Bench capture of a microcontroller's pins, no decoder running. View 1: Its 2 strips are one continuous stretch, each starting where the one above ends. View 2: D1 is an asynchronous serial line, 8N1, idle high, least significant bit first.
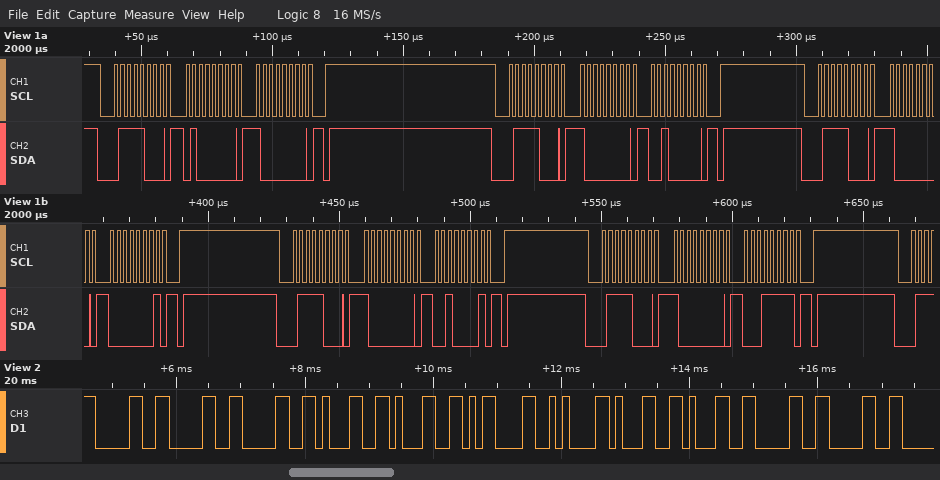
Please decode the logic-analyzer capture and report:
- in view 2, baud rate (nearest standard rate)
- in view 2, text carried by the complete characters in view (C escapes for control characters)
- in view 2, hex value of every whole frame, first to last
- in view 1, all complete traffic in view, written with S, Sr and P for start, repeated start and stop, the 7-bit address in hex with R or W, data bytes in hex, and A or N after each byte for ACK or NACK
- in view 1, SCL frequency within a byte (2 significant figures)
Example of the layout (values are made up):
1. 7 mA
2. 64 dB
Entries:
1. 9600 baud
2. "00011\r\n1100"
3. 30 30 30 31 31 0D 0A 31 31 30 30
4. S 3CW A 40 A 80 A P S 3CW A 80 A 20 A P S 3CW A 80 A 01 A P S 3CW A 80 A 21 A P S 3CW A 80 A 1F A P
5. 400 kHz
